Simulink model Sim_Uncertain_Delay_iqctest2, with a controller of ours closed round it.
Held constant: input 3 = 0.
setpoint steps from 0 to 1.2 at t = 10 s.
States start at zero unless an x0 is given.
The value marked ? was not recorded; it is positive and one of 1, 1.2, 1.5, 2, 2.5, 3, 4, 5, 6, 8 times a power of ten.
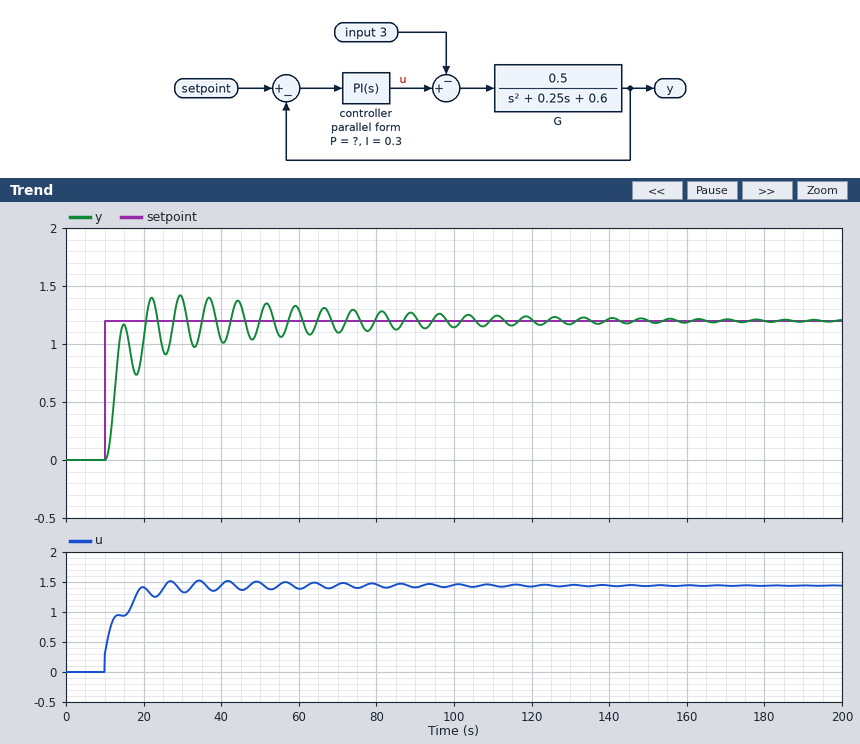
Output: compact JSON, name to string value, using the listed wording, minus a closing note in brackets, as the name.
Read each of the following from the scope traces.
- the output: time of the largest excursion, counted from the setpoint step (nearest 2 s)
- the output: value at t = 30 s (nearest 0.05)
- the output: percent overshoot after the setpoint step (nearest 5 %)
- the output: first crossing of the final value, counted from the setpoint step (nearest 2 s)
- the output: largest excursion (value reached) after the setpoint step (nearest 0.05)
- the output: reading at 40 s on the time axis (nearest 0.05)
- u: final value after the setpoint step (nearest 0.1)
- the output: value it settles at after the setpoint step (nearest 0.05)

{"the output: time of the largest excursion, counted from the setpoint step": "20 s", "the output: value at t = 30 s": "1.40", "the output: percent overshoot after the setpoint step": "20 %", "the output: first crossing of the final value, counted from the setpoint step": "10 s", "the output: largest excursion (value reached) after the setpoint step": "1.40", "the output: reading at 40 s on the time axis": "1.05", "u: final value after the setpoint step": "1.4", "the output: value it settles at after the setpoint step": "1.20"}
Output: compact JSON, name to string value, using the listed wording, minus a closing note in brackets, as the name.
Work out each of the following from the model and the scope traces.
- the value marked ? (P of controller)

{"the value marked ?": "0.25"}
